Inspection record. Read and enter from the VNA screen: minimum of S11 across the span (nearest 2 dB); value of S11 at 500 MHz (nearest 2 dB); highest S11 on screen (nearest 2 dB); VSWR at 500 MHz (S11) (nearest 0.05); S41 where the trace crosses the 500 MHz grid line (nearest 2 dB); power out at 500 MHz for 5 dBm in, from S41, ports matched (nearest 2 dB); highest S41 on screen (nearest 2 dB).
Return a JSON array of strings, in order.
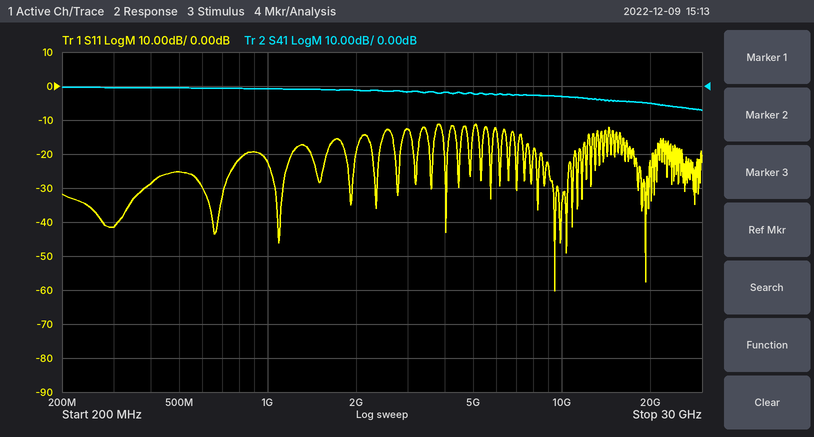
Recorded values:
["-60 dB", "-26 dB", "-12 dB", "1.10", "0 dB", "4 dBm", "0 dB"]
